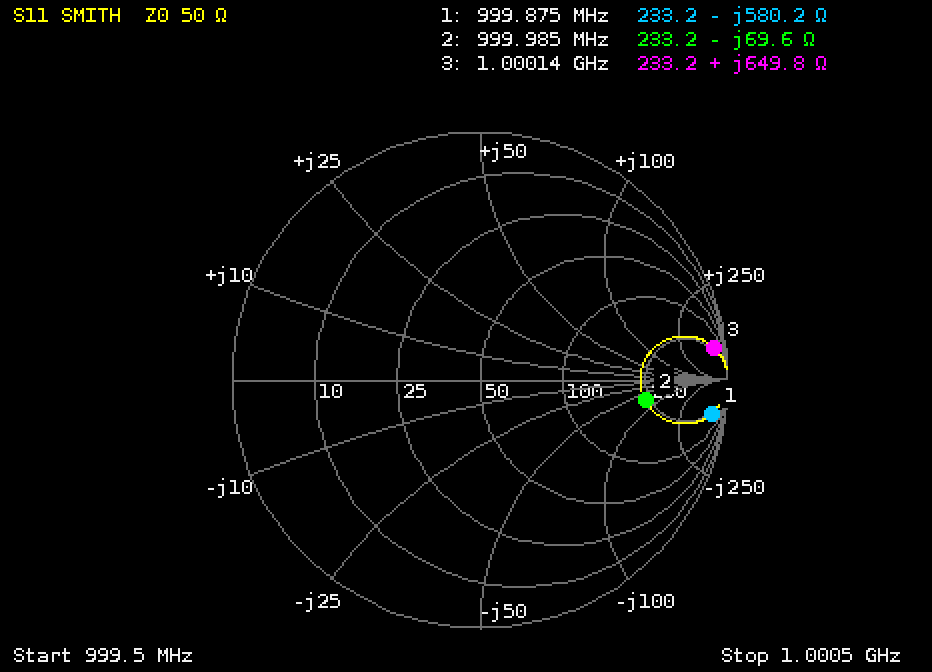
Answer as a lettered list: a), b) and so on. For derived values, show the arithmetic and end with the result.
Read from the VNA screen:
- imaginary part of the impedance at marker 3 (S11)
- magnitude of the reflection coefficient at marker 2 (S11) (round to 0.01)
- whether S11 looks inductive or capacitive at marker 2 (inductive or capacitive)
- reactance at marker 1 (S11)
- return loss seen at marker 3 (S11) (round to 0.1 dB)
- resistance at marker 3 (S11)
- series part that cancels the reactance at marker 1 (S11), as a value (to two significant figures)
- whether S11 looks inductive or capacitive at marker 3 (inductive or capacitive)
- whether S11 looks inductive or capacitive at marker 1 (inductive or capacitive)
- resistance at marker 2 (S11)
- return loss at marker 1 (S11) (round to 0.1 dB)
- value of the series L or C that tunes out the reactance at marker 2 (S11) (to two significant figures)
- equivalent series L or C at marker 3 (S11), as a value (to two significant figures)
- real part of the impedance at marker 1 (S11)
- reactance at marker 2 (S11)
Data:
a) +649.8 Ω
b) 0.67
c) capacitive
d) -580.2 Ω
e) 0.4 dB
f) 233.2 Ω
g) L = 580.2 Ω/(2π × 999.875 MHz) ≈ 92 nH
h) inductive
i) capacitive
j) 233.2 Ω
k) 0.5 dB
l) L = 69.6 Ω/(2π × 999.985 MHz) ≈ 11 nH
m) L = 649.8 Ω/(2π × 1.00014 GHz) ≈ 103 nH, so 100 nH to two significant figures
n) 233.2 Ω
o) -69.6 Ω
